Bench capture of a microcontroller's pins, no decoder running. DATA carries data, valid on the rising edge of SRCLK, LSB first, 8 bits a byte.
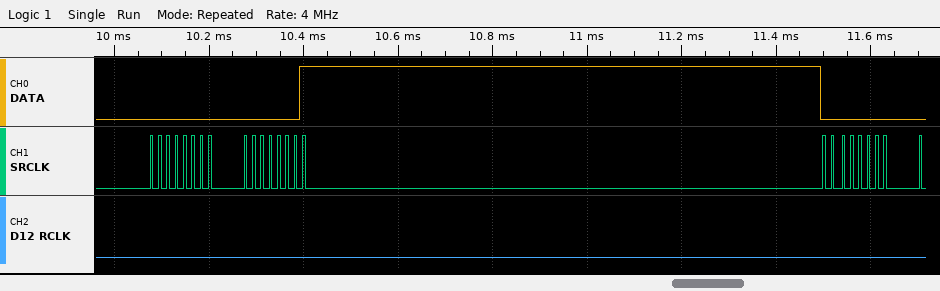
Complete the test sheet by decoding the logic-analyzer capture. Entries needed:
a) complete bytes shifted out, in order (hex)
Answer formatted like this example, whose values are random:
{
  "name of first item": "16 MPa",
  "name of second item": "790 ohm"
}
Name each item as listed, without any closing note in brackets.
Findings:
{
  "complete bytes shifted out, in order": "00 80 00"
}
